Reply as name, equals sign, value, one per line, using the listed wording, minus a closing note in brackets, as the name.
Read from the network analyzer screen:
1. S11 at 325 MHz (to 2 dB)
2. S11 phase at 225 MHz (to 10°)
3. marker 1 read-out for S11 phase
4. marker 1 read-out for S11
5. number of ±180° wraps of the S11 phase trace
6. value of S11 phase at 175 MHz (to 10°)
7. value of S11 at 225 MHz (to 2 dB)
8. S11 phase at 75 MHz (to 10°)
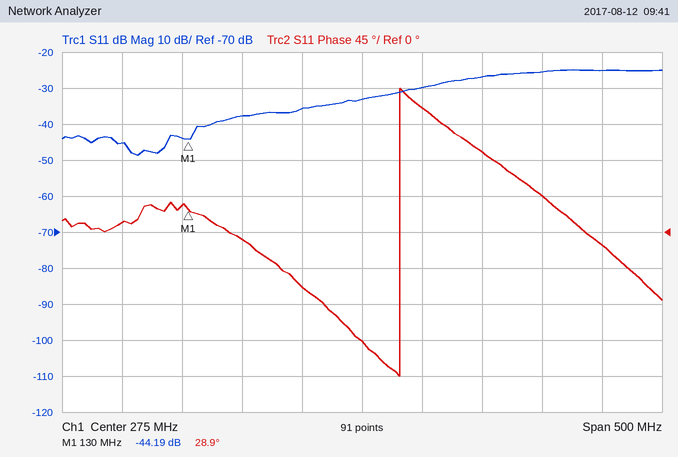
S11 at 325 MHz = -30 dB
S11 phase at 225 MHz = -70°
marker 1 read-out for S11 phase = 28.9°
marker 1 read-out for S11 = -44.19 dB
number of ±180° wraps of the S11 phase trace = 1
value of S11 phase at 175 MHz = -10°
value of S11 at 225 MHz = -36 dB
S11 phase at 75 MHz = 10°
